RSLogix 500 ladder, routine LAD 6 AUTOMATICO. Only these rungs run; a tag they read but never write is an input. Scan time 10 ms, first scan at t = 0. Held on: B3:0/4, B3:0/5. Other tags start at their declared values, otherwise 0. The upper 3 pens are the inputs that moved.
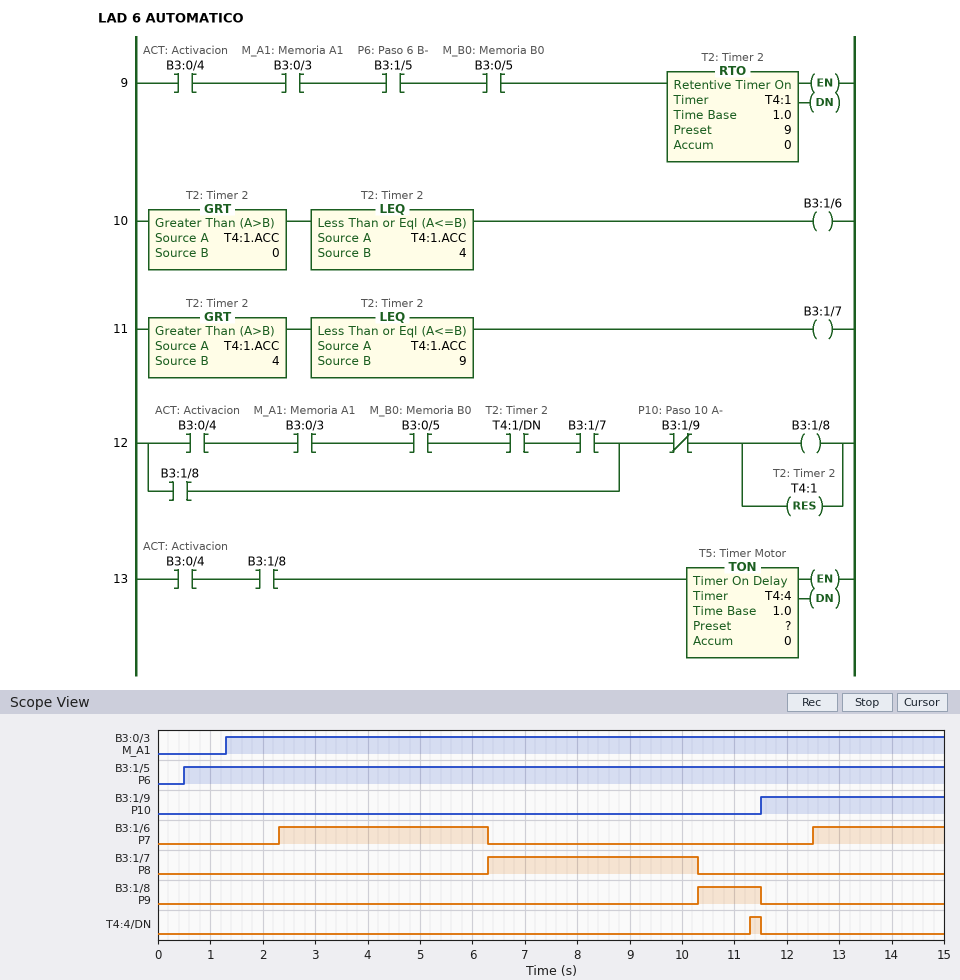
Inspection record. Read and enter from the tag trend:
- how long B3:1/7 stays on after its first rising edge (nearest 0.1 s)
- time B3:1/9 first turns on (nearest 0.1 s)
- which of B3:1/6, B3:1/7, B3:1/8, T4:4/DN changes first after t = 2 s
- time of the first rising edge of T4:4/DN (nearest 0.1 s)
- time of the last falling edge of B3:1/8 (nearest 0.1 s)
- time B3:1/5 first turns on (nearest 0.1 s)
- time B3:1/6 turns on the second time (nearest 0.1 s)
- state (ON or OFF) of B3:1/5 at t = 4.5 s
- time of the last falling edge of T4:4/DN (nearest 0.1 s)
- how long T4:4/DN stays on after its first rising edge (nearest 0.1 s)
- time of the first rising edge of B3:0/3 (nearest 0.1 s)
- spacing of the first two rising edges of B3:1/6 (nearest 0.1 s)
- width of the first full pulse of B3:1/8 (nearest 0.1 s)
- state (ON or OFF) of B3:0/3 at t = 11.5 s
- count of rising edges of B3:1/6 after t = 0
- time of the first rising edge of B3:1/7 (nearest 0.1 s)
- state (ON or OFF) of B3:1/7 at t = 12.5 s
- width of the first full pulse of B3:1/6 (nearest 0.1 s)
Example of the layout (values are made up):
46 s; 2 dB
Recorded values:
4.0 s; 11.5 s; B3:1/6; 11.3 s; 11.5 s; 0.5 s; 12.5 s; ON; 11.5 s; 0.2 s; 1.3 s; 10.2 s; 1.2 s; ON; 2; 6.3 s; OFF; 4.0 s
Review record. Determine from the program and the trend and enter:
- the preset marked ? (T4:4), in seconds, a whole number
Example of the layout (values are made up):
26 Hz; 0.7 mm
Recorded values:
1 s
